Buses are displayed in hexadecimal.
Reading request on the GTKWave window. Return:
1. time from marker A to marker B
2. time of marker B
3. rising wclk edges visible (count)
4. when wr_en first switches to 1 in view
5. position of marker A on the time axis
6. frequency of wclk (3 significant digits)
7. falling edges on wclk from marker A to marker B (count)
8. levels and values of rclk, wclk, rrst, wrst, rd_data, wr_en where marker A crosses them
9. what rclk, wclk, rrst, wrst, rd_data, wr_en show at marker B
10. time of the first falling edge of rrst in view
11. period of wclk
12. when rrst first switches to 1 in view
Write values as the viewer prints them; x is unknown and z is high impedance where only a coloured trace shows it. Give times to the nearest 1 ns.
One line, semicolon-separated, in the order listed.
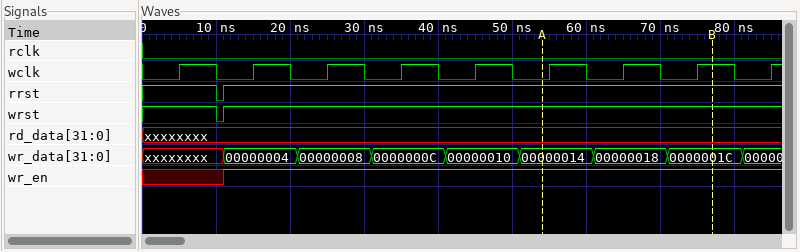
23 ns; 77 ns; 9; 11 ns; 54 ns; 100 MHz; 2; rclk=0, wclk=0, rrst=1, wrst=1, rd_data=xxxxxxxx, wr_en=1; rclk=0, wclk=1, rrst=1, wrst=1, rd_data=xxxxxxxx, wr_en=1; 10 ns; 10 ns; 11 ns
